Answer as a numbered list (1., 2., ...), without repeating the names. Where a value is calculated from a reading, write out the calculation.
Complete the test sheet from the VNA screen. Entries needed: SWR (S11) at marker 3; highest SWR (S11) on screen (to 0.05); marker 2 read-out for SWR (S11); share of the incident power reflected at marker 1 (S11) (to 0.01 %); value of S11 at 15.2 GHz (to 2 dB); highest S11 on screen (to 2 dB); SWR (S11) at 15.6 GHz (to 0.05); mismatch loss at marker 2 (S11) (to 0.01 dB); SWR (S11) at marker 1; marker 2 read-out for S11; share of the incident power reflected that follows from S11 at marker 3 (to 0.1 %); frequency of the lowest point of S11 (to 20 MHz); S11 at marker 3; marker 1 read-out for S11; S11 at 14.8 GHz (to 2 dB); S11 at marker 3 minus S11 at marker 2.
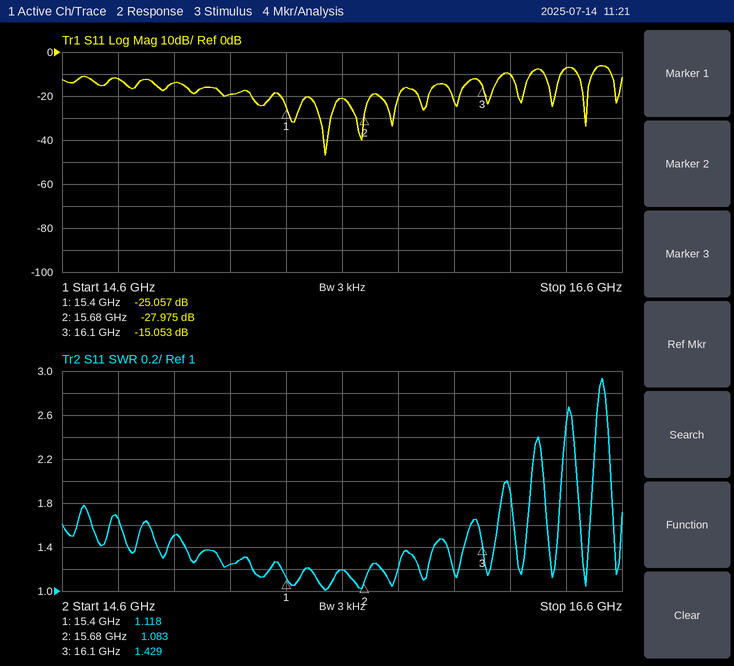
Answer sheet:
1. 1.429
2. 2.95
3. 1.083
4. 10^(-25.057/10) ≈ 0.31 %
5. -20 dB
6. -6 dB
7. 1.20
8. −10 log10(1 − 10^(-27.975/10)) ≈ 0.01 dB
9. 1.118
10. -27.975 dB
11. 10^(-15.053/10) ≈ 3.1 %
12. 15.54 GHz
13. -15.053 dB
14. -25.057 dB
15. -12 dB
16. -15.053 − (-27.975) = 12.922 dB
